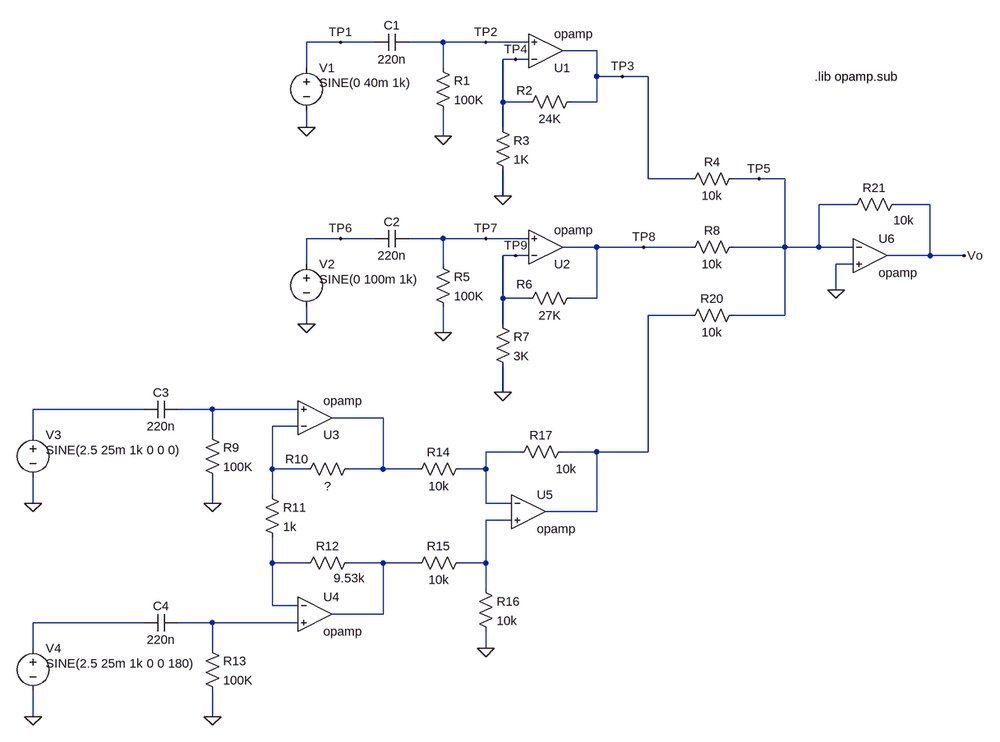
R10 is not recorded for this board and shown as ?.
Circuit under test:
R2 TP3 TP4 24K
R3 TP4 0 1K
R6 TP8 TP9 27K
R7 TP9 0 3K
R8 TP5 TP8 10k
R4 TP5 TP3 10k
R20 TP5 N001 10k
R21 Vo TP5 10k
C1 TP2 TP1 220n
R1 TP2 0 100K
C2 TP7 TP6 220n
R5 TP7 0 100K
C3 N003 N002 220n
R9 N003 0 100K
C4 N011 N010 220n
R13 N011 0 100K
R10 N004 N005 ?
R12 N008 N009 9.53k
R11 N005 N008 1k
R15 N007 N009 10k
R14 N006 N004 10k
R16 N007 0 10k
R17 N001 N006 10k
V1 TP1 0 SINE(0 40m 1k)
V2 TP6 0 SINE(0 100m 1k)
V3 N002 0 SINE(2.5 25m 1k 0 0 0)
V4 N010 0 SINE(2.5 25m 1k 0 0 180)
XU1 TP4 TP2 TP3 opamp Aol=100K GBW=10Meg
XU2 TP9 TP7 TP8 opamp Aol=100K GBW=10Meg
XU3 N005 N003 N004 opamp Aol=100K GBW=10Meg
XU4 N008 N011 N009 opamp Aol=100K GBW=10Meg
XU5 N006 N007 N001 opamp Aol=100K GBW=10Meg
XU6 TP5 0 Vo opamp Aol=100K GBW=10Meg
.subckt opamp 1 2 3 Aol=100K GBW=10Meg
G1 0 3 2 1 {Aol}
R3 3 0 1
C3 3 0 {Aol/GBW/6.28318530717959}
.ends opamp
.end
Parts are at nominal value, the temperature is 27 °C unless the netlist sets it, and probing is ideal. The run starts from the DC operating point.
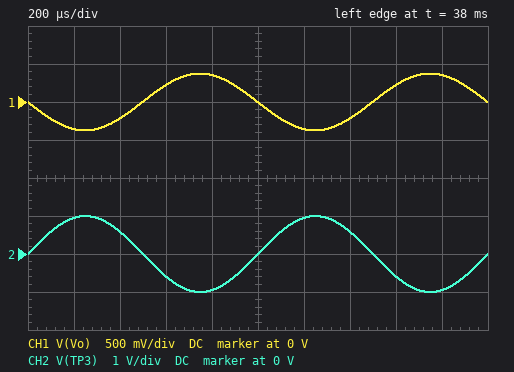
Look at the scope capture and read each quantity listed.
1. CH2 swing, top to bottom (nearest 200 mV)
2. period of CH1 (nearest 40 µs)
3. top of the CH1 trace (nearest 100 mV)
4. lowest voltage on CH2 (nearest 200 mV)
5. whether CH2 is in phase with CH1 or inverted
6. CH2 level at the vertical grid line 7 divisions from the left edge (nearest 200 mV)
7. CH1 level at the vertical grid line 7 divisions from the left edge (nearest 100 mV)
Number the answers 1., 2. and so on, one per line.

1. 2.0 V
2. 1.00 ms
3. 400 mV
4. -1.0 V
5. inverted
6. 600 mV
7. -200 mV
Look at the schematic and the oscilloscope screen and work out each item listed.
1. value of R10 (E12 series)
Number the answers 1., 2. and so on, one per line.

1. 22 kΩ
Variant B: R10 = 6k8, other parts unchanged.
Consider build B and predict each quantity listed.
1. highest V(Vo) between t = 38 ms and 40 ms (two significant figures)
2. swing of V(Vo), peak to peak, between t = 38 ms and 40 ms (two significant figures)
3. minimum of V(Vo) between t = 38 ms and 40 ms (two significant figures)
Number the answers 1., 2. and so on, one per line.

1. 1.1 V
2. 2.3 V
3. -1.1 V
